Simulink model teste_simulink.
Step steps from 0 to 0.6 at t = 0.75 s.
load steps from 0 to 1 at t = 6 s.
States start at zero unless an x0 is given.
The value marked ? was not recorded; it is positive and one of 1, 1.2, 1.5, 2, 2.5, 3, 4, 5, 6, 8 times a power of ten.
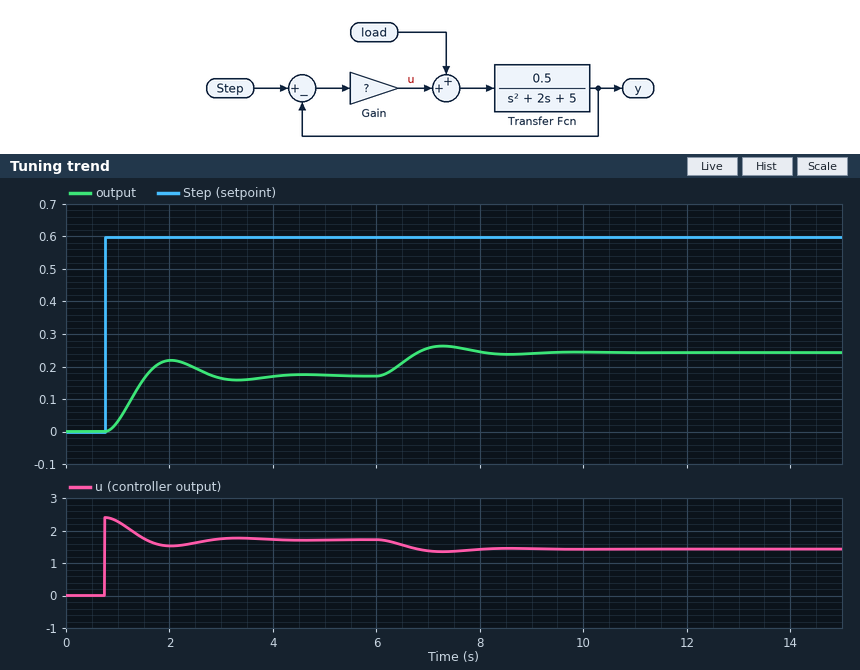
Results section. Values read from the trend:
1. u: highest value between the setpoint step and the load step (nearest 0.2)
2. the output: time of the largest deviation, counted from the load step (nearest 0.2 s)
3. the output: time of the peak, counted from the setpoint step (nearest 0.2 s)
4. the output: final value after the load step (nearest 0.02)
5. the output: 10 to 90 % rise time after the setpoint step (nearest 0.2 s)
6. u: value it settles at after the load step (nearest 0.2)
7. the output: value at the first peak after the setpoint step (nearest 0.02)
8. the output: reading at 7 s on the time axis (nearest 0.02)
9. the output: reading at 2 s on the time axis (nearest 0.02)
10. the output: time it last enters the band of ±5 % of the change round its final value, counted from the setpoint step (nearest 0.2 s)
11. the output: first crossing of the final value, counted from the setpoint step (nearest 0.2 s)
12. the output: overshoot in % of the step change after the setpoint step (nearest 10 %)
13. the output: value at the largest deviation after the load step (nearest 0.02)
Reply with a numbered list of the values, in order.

1. 2.4
2. 1.2 s
3. 1.2 s
4. 0.24
5. 0.6 s
6. 1.4
7. 0.22
8. 0.26
9. 0.22
10. 3.0 s
11. 0.8 s
12. 30 %
13. 0.26
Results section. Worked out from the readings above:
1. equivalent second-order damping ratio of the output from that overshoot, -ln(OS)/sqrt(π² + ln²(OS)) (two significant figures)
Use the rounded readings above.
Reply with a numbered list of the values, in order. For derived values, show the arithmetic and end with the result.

1. ln(0.3) = -1.204; 1.204 / sqrt(9.870 + 1.450) = 0.36
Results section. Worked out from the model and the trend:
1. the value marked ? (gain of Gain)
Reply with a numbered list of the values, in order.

1. 4
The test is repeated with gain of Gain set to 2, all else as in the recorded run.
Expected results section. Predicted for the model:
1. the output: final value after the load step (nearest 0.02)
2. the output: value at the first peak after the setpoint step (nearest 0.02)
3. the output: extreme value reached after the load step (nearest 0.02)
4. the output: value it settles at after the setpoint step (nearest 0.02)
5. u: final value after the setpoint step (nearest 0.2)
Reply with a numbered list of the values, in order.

1. 0.18
2. 0.12
3. 0.20
4. 0.10
5. 1.0
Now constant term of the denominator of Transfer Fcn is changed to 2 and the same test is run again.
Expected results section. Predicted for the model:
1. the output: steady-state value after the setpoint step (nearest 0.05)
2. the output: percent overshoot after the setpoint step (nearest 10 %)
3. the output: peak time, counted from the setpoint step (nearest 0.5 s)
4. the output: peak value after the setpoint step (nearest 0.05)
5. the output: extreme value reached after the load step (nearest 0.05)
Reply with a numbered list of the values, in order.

1. 0.30
2. 20 %
3. 2.0 s
4. 0.35
5. 0.45
